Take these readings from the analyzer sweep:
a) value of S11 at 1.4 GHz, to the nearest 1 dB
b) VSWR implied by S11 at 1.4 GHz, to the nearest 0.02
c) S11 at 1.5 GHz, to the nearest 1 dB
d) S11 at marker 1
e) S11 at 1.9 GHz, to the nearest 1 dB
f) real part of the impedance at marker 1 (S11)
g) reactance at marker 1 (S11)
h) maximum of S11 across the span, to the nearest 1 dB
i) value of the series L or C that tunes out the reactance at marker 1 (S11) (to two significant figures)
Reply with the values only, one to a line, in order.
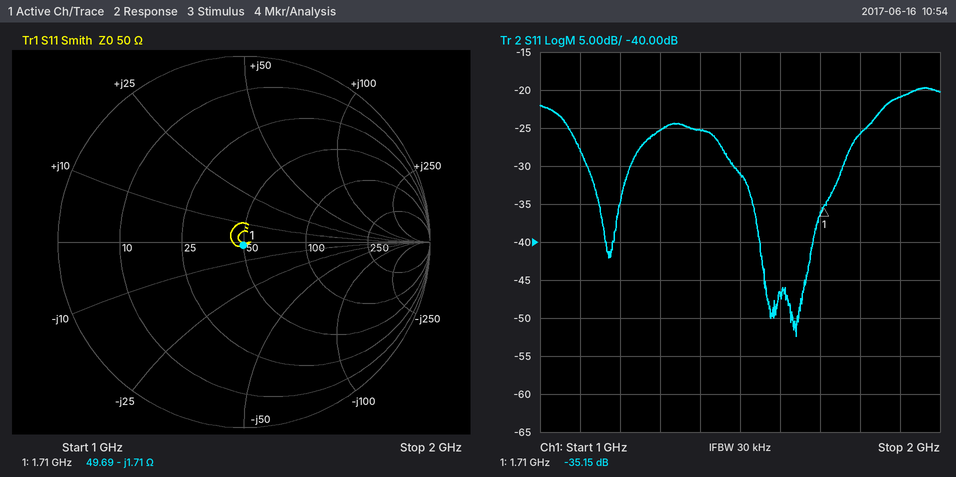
-25 dB
1.12
-31 dB
-35.15 dB
-21 dB
49.69 Ω
-1.71 Ω
-20 dB
160 pH
